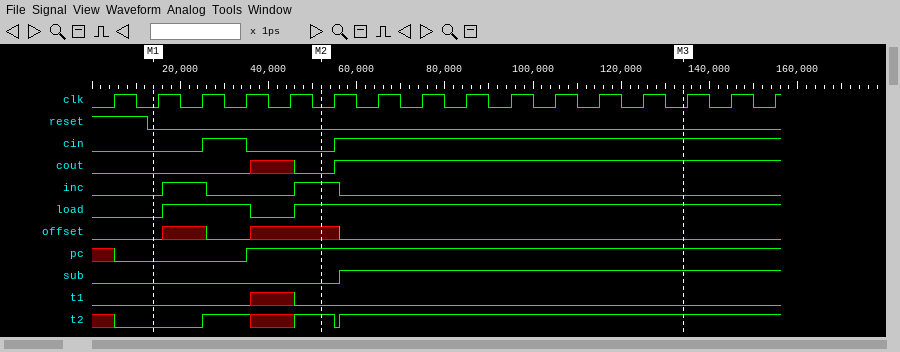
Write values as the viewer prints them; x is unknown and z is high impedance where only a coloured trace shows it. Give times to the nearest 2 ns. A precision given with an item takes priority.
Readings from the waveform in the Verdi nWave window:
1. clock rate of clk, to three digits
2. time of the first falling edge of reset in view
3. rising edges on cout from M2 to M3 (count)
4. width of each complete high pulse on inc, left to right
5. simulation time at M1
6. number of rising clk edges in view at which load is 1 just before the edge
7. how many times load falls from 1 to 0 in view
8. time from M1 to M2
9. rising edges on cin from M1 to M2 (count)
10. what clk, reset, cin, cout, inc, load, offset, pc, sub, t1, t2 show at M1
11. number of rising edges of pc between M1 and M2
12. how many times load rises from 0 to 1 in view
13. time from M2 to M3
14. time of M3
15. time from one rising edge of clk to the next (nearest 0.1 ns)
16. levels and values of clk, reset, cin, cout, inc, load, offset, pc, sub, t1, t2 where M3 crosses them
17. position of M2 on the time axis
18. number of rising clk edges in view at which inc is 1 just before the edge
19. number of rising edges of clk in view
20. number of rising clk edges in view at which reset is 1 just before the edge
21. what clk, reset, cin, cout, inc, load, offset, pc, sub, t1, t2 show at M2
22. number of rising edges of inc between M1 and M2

100 MHz
12 ns
1
10 ns, 10 ns
14 ns
13
1
38 ns
1
clk=0, reset=0, cin=0, cout=0, inc=0, load=0, offset=0, pc=0, sub=0, t1=0, t2=0
1
2
82 ns
134 ns
10 ns
clk=0, reset=0, cin=1, cout=1, inc=0, load=1, offset=0, pc=1, sub=1, t1=0, t2=1
52 ns
2
16
1
clk=0, reset=0, cin=0, cout=0, inc=1, load=1, offset=x, pc=1, sub=0, t1=0, t2=1
2
